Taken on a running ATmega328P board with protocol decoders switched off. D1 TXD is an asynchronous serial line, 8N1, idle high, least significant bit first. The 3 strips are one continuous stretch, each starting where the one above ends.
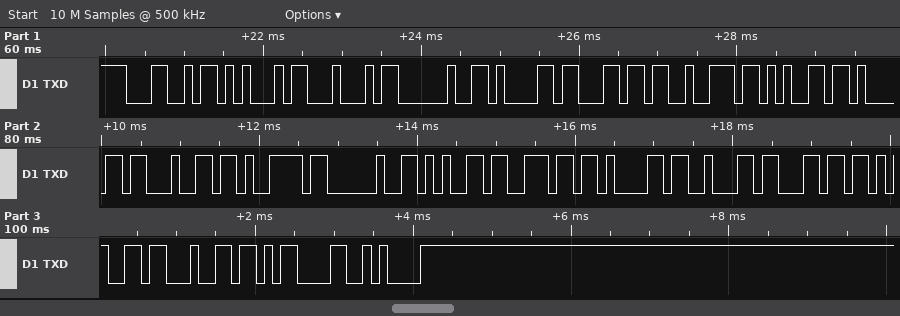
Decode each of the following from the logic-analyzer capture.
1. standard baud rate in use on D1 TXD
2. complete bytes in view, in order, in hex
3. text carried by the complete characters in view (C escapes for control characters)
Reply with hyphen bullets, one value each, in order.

- 9600 baud
- 4C 45 44 20 61 6C 72 65 61 64 79 20 65 6E 61 62 6C 65 64 0D 0A
- "LED already enabled\r\n"
